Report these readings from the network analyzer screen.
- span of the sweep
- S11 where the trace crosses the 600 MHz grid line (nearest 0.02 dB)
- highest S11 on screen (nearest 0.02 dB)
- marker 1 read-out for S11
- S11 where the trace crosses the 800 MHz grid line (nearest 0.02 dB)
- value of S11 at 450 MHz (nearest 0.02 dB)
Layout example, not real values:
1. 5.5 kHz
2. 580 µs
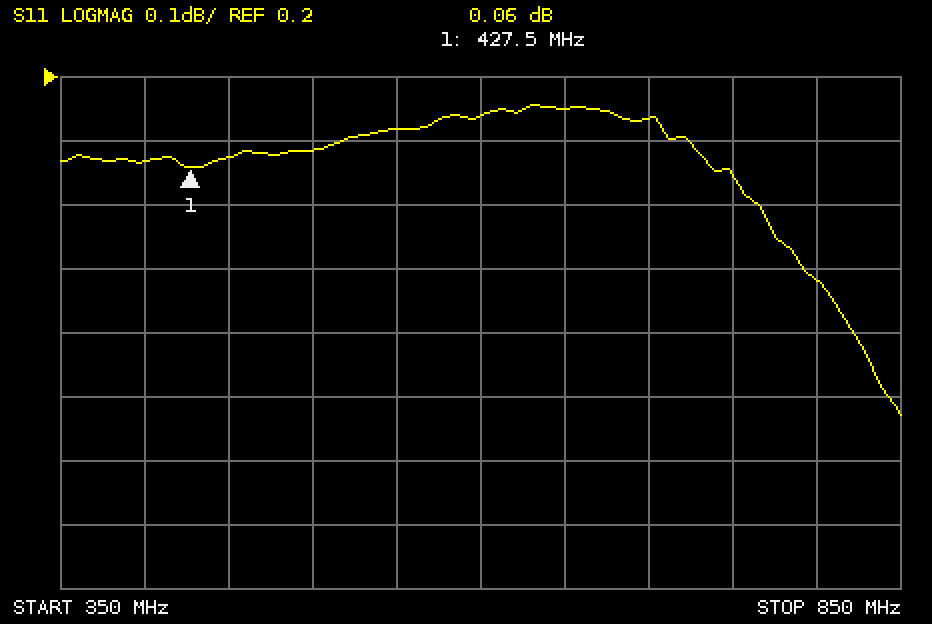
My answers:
1. 500 MHz
2. 0.14 dB
3. 0.16 dB
4. 0.06 dB
5. -0.12 dB
6. 0.08 dB
